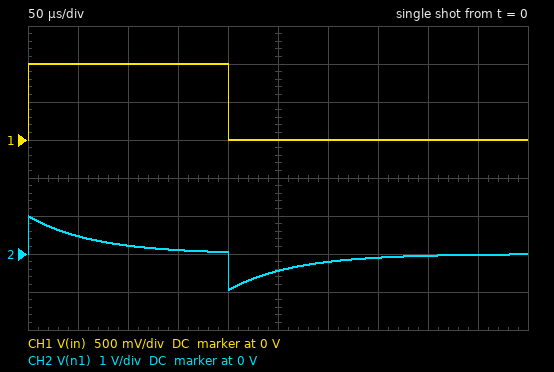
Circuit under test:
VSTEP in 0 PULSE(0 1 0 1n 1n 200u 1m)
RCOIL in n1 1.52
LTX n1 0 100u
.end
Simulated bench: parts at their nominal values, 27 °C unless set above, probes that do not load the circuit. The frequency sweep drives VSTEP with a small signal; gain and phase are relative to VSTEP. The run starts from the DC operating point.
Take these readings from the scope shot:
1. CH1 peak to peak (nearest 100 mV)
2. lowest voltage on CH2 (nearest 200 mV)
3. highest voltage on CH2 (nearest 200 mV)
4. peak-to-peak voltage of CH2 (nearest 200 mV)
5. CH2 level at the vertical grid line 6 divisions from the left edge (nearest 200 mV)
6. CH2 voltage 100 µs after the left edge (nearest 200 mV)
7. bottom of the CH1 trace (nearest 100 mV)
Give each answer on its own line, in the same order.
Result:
1.0 V
-1.0 V
1.0 V
2.0 V
-200 mV
200 mV
0 V
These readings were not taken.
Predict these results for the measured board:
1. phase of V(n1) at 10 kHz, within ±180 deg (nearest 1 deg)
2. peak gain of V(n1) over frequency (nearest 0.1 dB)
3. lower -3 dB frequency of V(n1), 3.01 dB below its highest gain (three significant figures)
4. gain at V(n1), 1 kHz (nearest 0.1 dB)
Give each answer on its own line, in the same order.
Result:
14 deg
0 dB
2.42 kHz
-8.4 dB
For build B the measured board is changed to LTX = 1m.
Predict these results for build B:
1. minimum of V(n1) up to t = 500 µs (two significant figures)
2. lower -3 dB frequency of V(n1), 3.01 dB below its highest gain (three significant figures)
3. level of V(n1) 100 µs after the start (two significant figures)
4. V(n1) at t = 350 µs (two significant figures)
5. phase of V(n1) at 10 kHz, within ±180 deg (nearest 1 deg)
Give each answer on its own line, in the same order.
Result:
-260 mV
242 Hz
860 mV
-210 mV
1 deg
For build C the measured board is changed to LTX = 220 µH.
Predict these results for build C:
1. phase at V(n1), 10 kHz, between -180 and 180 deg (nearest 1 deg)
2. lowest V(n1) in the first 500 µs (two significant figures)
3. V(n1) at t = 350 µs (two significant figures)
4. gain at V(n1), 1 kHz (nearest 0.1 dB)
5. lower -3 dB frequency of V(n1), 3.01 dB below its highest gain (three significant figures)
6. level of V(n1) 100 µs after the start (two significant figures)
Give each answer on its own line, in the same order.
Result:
6 deg
-750 mV
-270 mV
-3.4 dB
1.10 kHz
500 mV
